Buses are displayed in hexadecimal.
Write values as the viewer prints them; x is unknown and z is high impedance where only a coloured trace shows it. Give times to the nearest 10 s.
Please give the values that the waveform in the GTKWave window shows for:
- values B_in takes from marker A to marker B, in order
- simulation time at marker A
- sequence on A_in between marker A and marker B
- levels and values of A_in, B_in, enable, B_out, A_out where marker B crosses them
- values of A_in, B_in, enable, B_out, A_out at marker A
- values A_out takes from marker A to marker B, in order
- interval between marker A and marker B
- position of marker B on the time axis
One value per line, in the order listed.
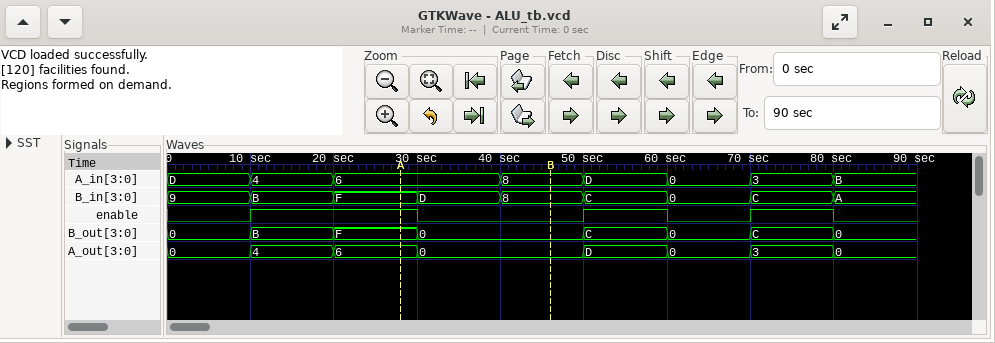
F, D, 8
30 s
6, 8
A_in=8, B_in=8, enable=0, B_out=0, A_out=0
A_in=6, B_in=F, enable=1, B_out=F, A_out=6
6, 0
20 s
50 s
